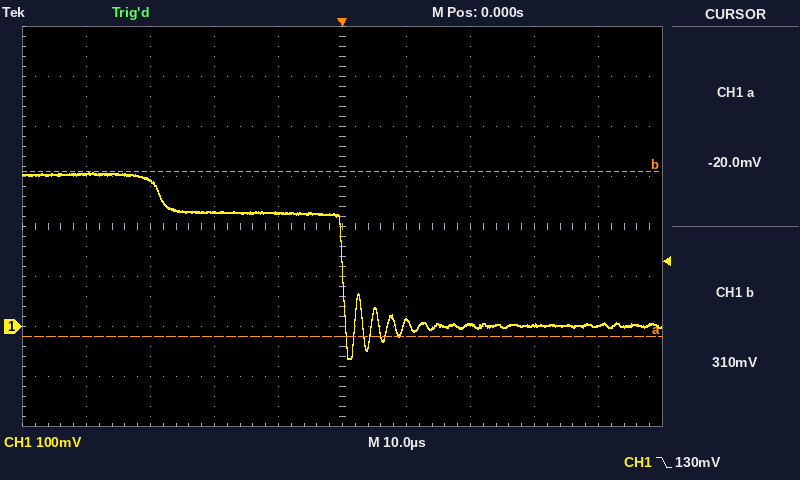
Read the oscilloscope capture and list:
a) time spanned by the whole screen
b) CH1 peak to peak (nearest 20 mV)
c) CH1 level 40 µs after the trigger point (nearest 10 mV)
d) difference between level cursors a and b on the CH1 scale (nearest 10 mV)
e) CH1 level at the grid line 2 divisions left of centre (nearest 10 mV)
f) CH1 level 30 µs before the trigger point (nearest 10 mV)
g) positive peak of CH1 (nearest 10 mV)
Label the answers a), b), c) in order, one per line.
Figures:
a) 100 µs
b) 380 mV
c) 0 mV
d) 330 mV
e) 230 mV
f) 290 mV
g) 310 mV
